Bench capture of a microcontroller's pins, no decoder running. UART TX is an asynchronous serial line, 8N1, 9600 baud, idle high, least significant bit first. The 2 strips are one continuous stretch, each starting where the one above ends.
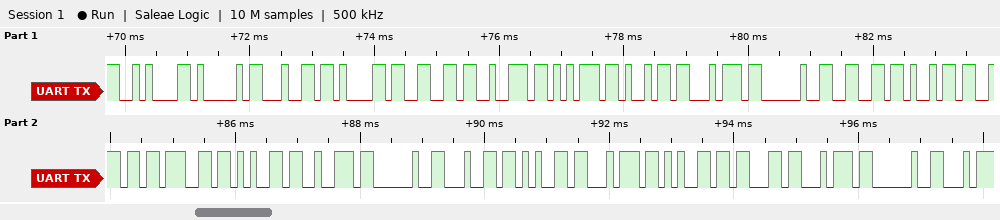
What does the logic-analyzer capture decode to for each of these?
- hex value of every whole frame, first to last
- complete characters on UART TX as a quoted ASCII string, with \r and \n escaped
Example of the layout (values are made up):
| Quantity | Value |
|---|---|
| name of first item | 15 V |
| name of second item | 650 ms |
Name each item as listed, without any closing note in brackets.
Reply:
| Quantity | Value |
|---|---|
| hex value of every whole frame, first to last | 0A 41 64 61 66 72 75 69 74 20 66 69 6E 67 65 72 20 64 65 74 65 63 74 20 |
| complete characters on UART TX as a quoted ASCII string, with \r and \n escaped | "\nAdafruit finger detect " |
